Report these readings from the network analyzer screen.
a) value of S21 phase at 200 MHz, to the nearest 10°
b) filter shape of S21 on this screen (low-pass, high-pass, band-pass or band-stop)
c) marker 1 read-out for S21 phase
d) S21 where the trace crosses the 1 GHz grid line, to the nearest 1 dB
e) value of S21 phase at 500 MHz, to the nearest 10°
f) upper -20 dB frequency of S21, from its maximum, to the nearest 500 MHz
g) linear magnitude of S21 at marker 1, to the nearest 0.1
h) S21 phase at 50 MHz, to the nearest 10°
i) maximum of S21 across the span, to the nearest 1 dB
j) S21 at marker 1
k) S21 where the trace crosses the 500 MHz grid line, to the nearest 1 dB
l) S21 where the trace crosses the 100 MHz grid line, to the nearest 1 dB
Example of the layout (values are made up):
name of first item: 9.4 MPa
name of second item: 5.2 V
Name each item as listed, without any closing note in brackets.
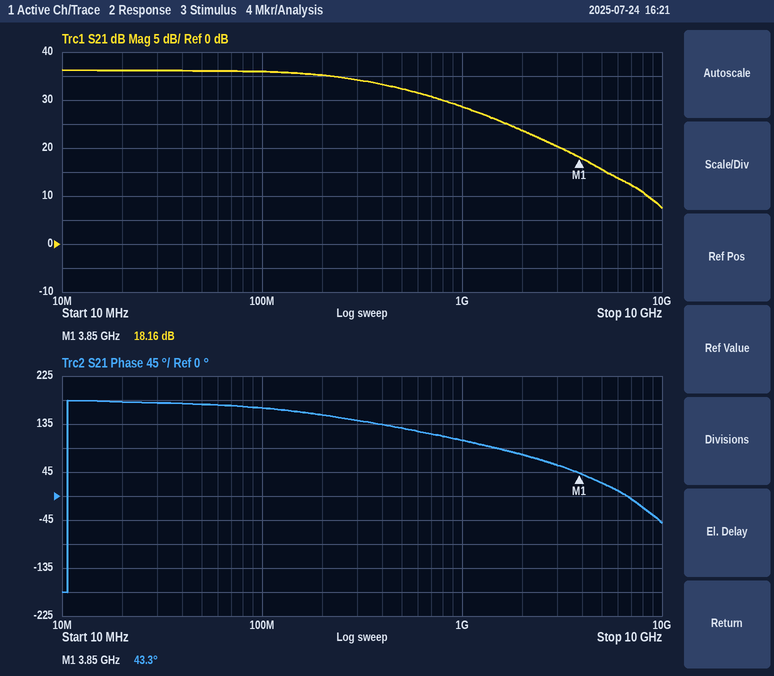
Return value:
value of S21 phase at 200 MHz, to the nearest 10°: 150°
filter shape of S21 on this screen: low-pass
marker 1 read-out for S21 phase: 43.3°
S21 where the trace crosses the 1 GHz grid line, to the nearest 1 dB: 29 dB
value of S21 phase at 500 MHz, to the nearest 10°: 130°
upper -20 dB frequency of S21, from its maximum, to the nearest 500 MHz: 4.5 GHz
linear magnitude of S21 at marker 1, to the nearest 0.1: 8.1
S21 phase at 50 MHz, to the nearest 10°: 170°
maximum of S21 across the span, to the nearest 1 dB: 36 dB
S21 at marker 1: 18.16 dB
S21 where the trace crosses the 500 MHz grid line, to the nearest 1 dB: 32 dB
S21 where the trace crosses the 100 MHz grid line, to the nearest 1 dB: 36 dB
